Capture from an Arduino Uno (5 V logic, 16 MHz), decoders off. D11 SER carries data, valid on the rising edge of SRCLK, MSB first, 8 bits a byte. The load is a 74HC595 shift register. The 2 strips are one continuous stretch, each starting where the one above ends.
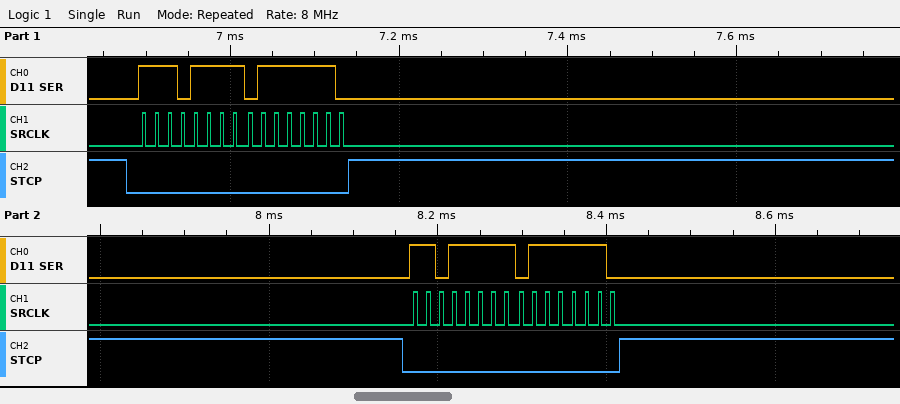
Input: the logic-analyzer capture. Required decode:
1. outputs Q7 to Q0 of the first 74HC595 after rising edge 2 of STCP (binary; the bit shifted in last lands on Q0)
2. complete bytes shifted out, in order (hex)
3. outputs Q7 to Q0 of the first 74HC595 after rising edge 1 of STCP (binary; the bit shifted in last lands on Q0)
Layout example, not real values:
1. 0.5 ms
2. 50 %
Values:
1. 01111110
2. EF 7E DF 7E
3. 01111110
